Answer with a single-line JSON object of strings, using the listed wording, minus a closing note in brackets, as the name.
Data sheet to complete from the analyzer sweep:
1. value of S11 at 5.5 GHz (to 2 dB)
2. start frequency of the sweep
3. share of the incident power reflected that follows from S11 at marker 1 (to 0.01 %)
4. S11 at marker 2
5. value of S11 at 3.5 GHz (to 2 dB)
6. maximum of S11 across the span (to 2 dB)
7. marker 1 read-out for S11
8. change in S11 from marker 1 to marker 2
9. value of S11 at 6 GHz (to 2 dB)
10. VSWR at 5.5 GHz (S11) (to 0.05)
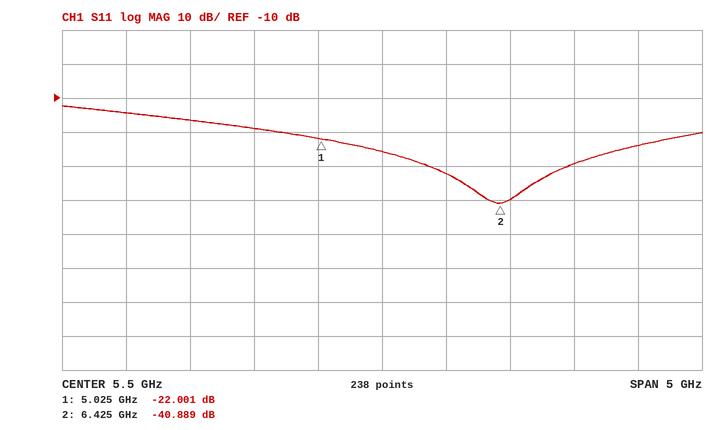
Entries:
{"value of S11 at 5.5 GHz": "-26 dB", "start frequency of the sweep": "3 GHz", "share of the incident power reflected that follows from S11 at marker 1": "0.63 %", "S11 at marker 2": "-40.889 dB", "value of S11 at 3.5 GHz": "-14 dB", "maximum of S11 across the span": "-12 dB", "marker 1 read-out for S11": "-22.001 dB", "change in S11 from marker 1 to marker 2": "-18.888 dB", "value of S11 at 6 GHz": "-32 dB", "VSWR at 5.5 GHz (S11)": "1.10"}
